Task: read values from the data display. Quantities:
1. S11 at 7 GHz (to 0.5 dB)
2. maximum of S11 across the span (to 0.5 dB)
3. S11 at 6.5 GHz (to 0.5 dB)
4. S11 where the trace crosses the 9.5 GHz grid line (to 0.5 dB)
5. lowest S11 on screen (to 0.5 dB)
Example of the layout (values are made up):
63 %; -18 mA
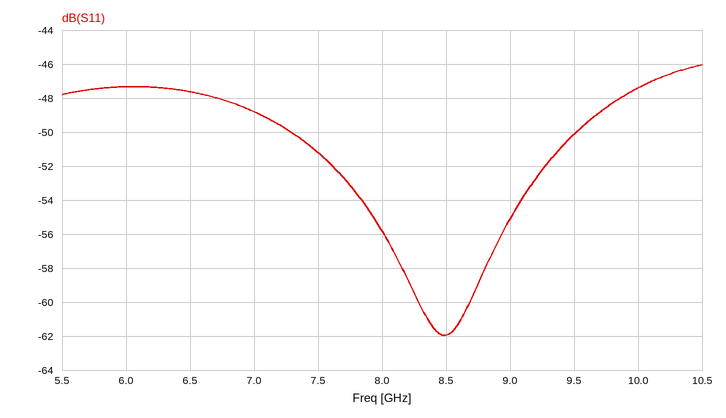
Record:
-49.0 dB; -46.0 dB; -47.5 dB; -50.0 dB; -62.0 dB
